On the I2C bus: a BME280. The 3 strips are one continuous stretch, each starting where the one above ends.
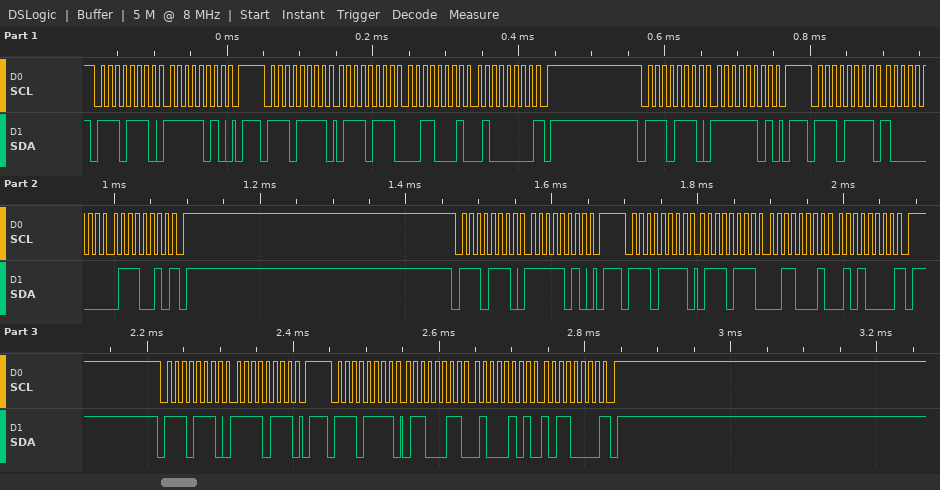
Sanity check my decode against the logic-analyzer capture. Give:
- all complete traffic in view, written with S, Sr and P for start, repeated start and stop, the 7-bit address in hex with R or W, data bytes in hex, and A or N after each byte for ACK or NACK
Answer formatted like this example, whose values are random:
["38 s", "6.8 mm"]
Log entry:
["S 77W A FA A P S 77R A 77 A 31 A 40 N P S 77W A FD A P S 77R A 80 A 72 N P S 77W A FA A P S 77R A 77 A 31 A 50 N P S 77W A F7 A P S 77R A 63 A 45 A B0 N P"]
